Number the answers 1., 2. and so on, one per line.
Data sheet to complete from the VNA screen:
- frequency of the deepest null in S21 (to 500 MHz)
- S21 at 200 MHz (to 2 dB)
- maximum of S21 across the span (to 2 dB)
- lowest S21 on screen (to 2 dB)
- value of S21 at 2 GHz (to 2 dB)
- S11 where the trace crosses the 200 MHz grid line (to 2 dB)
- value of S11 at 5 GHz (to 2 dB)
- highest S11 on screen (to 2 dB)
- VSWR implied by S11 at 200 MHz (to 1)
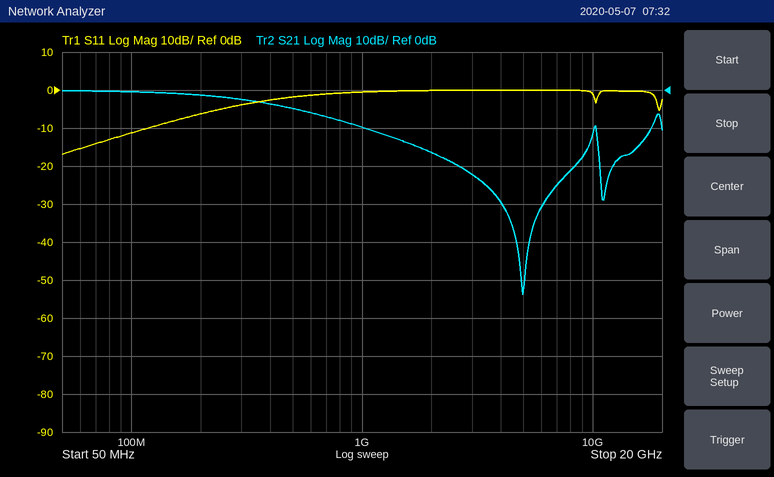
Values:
1. 5.0 GHz
2. -2 dB
3. 0 dB
4. -54 dB
5. -16 dB
6. -6 dB
7. 0 dB
8. 0 dB
9. 3
